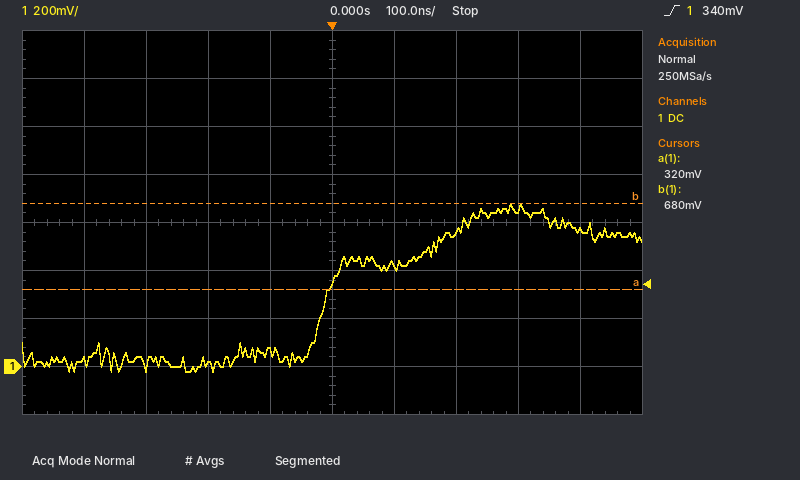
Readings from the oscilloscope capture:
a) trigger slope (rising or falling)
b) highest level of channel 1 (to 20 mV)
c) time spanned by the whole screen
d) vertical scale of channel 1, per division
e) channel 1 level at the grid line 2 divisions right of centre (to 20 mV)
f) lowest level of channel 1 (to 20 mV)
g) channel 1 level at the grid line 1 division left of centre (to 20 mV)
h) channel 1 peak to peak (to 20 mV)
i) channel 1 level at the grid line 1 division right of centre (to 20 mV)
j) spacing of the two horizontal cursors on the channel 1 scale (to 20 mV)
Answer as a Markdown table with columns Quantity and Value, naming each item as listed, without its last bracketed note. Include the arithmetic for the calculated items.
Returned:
| Quantity | Value |
|---|---|
| trigger slope | rising |
| highest level of channel 1 | 680 mV |
| time spanned by the whole screen | 1 µs |
| vertical scale of channel 1, per division | 200 mV |
| channel 1 level at the grid line 2 divisions right of centre | 560 mV |
| lowest level of channel 1 | -20 mV |
| channel 1 level at the grid line 1 division left of centre | 60 mV |
| channel 1 peak to peak | 680 mV − (-20 mV) = 700 mV |
| channel 1 level at the grid line 1 division right of centre | 420 mV |
| spacing of the two horizontal cursors on the channel 1 scale | 360 mV |
